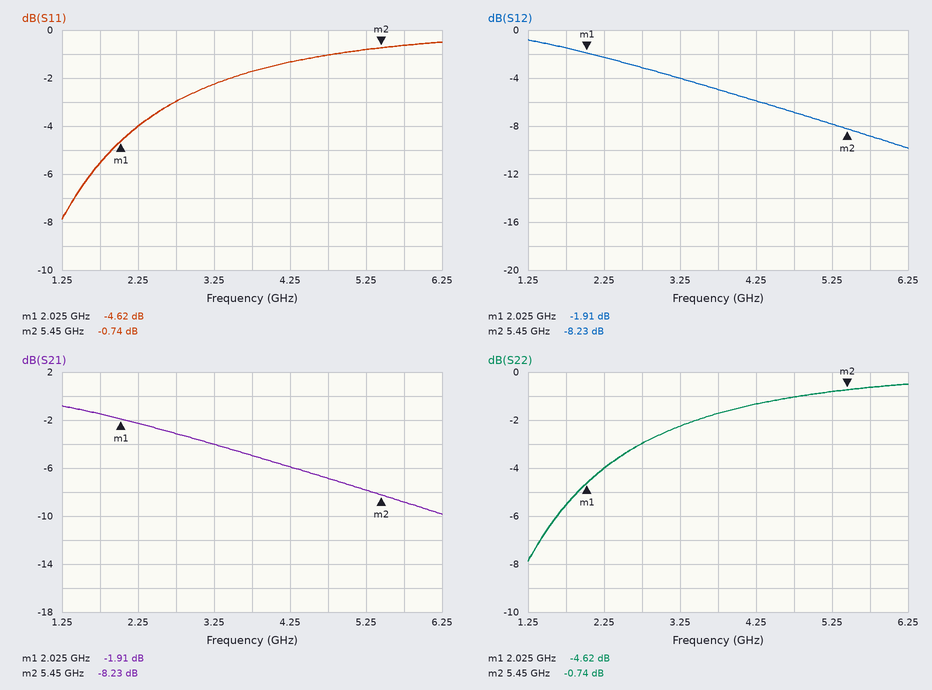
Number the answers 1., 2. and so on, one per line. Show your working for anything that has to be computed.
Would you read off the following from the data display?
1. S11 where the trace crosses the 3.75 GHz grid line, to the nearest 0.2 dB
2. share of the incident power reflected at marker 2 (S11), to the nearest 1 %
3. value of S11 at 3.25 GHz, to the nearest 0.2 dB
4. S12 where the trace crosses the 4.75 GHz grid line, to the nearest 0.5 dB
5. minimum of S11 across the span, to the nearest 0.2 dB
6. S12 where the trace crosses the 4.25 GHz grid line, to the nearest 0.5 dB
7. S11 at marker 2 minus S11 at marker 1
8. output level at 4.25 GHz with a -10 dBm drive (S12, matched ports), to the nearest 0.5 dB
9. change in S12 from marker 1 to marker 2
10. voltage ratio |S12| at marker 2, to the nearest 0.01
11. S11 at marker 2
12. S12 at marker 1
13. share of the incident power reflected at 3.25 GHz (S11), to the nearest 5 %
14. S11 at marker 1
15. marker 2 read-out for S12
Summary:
1. -1.8 dB
2. 10^(-0.74/10) ≈ 84 %
3. -2.2 dB
4. -7.0 dB
5. -7.8 dB
6. -6.0 dB
7. -0.74 − (-4.62) = 3.88 dB
8. -10 dBm + (-6.0 dB) = -16.0 dBm
9. -8.23 − (-1.91) = -6.32 dB
10. 10^(-8.23/20) ≈ 0.39
11. -0.74 dB
12. -1.91 dB
13. 10^(-2.2/10) ≈ 60 %
14. -4.62 dB
15. -8.23 dB
